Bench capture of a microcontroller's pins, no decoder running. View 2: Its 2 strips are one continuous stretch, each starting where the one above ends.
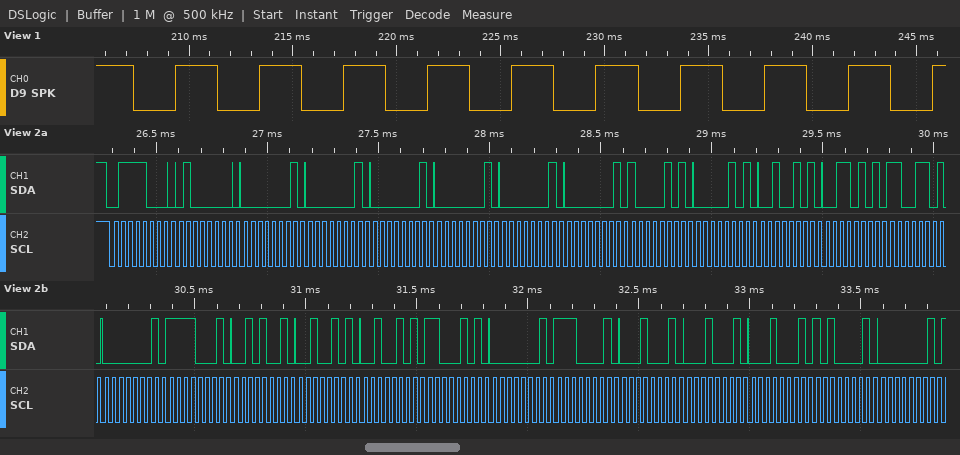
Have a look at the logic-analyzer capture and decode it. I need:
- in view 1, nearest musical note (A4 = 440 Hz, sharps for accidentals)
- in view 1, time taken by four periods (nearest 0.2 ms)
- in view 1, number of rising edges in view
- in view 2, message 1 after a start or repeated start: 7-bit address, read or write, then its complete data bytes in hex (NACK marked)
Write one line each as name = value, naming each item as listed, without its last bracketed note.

in view 1, nearest musical note = B3
in view 1, time taken by four periods = 16.2 ms
in view 1, number of rising edges in view = 10
in view 2, message 1 after a start or repeated start: 7-bit address, read or write, then its complete data bytes in hex = 0x3C write: 40 01 01 01 01 01 01 85 05 25 35 CD 01 F1 29 25 25 C5 01 E1 11 11 11 A1 01
